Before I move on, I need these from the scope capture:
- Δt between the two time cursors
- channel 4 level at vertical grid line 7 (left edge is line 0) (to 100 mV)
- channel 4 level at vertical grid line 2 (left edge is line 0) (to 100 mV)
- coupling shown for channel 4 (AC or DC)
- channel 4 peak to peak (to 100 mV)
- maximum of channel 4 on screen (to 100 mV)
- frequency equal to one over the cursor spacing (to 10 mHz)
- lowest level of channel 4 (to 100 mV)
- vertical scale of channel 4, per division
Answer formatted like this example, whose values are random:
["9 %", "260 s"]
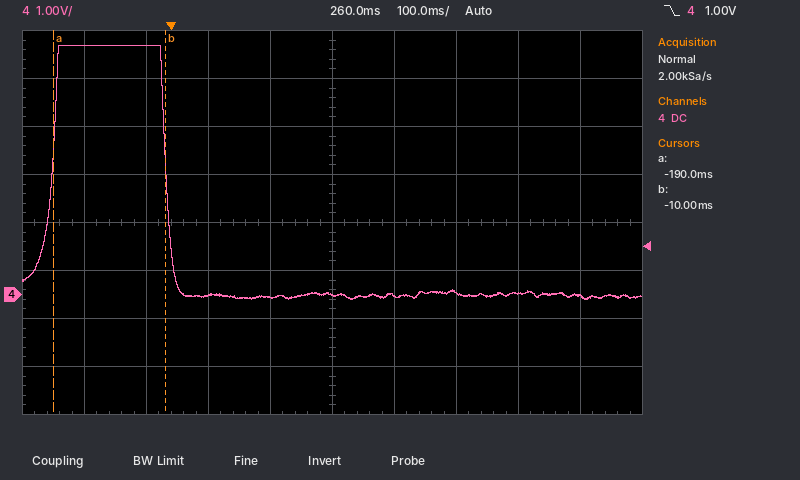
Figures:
["180 ms", "0.0 V", "5.2 V", "DC", "5.3 V", "5.2 V", "5.56 Hz", "-100 mV", "1 V"]
